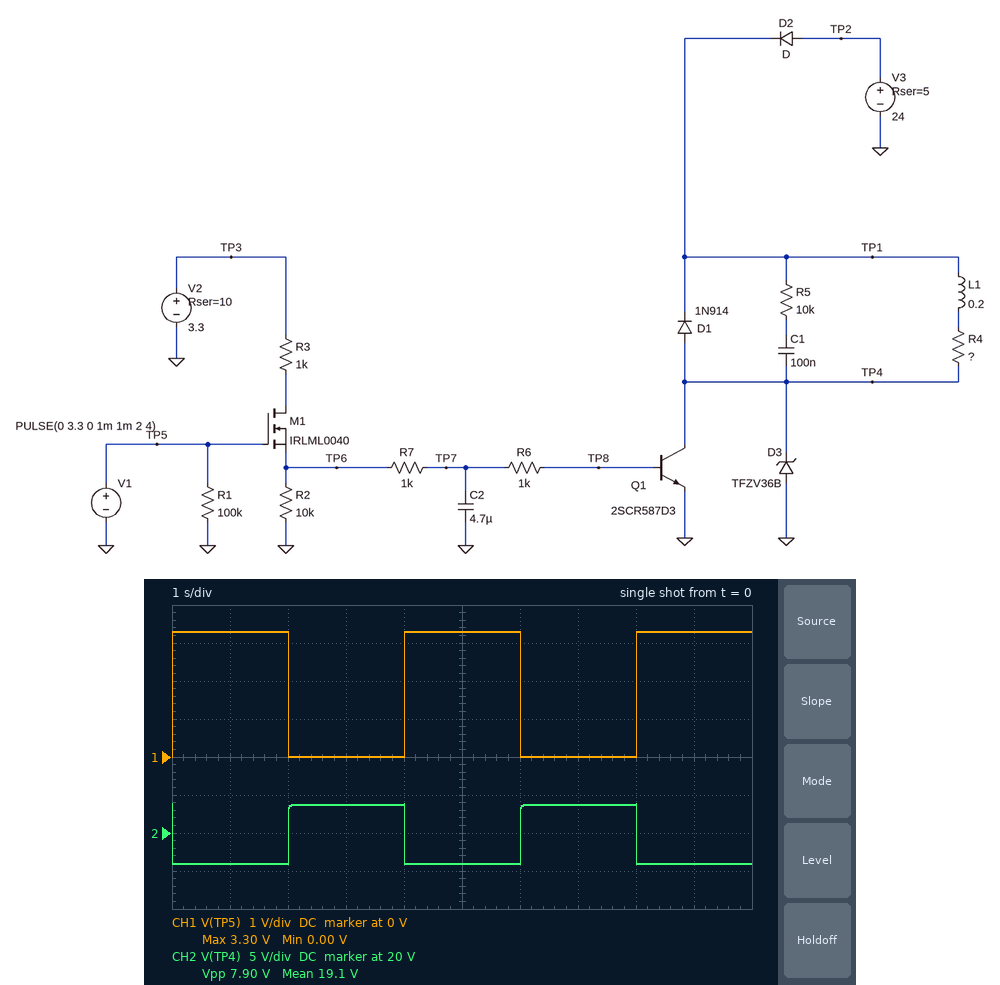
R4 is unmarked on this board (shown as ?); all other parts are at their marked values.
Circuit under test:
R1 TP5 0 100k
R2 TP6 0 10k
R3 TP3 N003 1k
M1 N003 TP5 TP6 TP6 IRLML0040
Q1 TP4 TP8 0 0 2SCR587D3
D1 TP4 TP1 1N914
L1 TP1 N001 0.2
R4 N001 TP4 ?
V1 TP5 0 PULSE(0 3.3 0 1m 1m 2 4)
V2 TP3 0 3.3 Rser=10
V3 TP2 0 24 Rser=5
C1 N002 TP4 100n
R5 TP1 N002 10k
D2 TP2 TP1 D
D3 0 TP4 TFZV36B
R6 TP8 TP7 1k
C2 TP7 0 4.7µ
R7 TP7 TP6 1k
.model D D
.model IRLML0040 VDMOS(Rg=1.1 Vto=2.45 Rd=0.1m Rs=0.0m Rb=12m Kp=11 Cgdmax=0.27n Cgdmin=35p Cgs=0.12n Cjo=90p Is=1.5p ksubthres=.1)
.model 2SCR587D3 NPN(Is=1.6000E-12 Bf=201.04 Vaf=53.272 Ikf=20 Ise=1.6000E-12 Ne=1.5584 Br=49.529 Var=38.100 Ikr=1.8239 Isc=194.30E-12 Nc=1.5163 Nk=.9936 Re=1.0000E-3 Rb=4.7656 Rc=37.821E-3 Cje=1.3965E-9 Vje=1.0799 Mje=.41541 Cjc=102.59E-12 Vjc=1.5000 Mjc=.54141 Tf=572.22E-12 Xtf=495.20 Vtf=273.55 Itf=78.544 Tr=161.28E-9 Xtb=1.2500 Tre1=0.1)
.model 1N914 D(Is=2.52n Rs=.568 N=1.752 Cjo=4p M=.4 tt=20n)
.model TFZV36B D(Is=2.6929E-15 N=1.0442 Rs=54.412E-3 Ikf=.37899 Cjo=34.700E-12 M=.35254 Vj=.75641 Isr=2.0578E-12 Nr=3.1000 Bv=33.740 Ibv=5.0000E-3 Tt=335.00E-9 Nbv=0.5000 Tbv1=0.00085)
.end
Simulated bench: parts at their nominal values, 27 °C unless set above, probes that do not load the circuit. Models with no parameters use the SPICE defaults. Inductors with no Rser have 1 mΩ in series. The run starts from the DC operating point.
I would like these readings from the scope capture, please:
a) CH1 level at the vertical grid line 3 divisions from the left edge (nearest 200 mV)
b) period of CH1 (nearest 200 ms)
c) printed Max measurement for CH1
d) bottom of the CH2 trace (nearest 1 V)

0 V
4.0 s
3.30 V
16 V
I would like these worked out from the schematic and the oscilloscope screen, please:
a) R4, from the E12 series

120 Ω
